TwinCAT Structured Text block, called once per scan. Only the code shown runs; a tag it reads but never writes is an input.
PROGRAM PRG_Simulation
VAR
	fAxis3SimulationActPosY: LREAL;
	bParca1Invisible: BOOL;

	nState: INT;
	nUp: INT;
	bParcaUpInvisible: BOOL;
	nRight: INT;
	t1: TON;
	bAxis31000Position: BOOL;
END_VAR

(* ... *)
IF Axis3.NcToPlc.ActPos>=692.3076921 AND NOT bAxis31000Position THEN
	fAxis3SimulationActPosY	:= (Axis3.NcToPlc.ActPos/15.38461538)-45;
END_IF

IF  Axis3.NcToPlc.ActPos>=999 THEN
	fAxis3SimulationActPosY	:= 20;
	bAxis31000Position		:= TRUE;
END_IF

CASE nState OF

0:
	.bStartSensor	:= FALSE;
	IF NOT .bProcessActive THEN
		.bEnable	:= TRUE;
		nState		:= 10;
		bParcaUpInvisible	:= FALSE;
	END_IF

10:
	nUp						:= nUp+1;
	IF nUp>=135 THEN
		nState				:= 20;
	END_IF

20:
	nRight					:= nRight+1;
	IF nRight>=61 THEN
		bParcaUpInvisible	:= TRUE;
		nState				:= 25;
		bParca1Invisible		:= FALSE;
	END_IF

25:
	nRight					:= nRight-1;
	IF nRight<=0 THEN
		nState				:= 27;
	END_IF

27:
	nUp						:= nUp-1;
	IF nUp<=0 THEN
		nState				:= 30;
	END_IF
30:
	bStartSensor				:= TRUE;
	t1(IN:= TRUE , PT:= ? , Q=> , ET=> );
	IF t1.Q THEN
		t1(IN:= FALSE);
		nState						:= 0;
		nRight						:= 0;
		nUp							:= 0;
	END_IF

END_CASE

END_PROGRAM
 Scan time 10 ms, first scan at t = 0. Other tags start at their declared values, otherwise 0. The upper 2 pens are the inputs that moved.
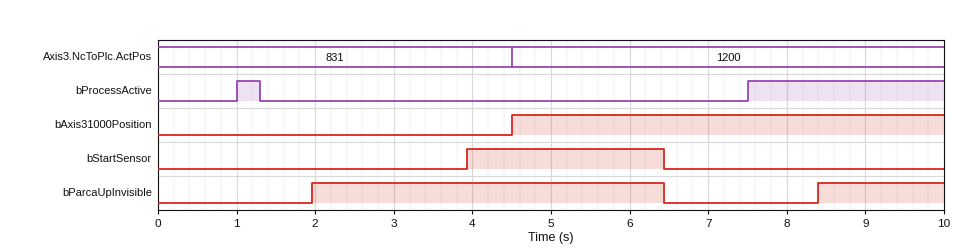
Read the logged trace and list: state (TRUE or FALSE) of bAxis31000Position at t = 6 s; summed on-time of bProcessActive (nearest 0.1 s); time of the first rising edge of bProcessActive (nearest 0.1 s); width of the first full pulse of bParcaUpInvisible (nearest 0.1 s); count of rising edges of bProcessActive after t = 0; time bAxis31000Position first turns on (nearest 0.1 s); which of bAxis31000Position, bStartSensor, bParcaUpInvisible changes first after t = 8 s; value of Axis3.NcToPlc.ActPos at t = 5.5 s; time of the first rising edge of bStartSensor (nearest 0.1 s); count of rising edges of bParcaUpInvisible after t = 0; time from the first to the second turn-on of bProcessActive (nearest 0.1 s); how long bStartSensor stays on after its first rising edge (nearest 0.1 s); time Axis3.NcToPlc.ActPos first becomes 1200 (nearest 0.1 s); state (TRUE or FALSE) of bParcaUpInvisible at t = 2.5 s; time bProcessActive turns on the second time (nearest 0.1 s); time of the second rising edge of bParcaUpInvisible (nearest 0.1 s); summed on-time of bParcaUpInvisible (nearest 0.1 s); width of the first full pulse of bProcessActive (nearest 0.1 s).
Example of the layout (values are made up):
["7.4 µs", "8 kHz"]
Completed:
["TRUE", "2.8 s", "1.0 s", "4.5 s", "2", "4.5 s", "bParcaUpInvisible", "1200", "3.9 s", "2", "6.5 s", "2.5 s", "4.5 s", "TRUE", "7.5 s", "8.4 s", "6.1 s", "0.3 s"]
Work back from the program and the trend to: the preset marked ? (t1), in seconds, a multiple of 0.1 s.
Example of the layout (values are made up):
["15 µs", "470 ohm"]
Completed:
["2.5 s"]
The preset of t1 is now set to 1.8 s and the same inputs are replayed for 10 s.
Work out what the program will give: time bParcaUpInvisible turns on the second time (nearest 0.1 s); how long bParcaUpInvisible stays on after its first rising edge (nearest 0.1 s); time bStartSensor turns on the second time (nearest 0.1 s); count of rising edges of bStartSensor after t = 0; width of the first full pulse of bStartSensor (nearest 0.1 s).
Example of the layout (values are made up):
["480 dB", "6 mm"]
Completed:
["7.7 s", "3.8 s", "9.7 s", "2", "1.8 s"]
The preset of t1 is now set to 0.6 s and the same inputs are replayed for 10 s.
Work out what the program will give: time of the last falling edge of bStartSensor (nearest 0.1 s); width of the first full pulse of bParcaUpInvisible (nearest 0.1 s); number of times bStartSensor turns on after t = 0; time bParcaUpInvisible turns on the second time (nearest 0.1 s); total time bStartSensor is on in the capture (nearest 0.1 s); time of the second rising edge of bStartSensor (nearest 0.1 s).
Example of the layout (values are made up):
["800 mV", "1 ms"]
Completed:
["9.1 s", "2.6 s", "2", "6.5 s", "1.2 s", "8.5 s"]
